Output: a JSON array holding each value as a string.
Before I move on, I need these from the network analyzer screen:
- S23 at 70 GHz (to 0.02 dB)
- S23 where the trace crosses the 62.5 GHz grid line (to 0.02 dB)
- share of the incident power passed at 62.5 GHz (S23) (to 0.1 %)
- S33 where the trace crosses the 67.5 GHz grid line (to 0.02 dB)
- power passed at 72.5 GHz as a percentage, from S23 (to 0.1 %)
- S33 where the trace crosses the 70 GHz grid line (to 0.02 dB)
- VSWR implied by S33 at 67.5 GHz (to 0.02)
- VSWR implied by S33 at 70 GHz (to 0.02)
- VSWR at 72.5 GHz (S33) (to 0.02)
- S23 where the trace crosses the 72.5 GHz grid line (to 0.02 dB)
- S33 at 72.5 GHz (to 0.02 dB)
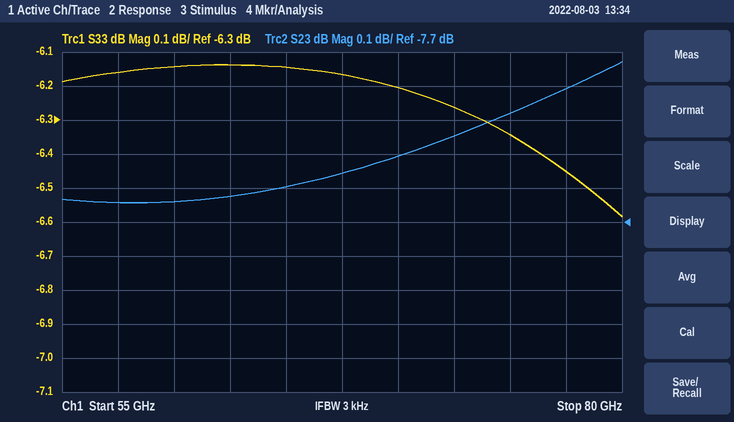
["-7.50 dB", "-7.62 dB", "17.3 %", "-6.16 dB", "18.0 %", "-6.20 dB", "2.94", "2.92", "2.90", "-7.44 dB", "-6.26 dB"]
